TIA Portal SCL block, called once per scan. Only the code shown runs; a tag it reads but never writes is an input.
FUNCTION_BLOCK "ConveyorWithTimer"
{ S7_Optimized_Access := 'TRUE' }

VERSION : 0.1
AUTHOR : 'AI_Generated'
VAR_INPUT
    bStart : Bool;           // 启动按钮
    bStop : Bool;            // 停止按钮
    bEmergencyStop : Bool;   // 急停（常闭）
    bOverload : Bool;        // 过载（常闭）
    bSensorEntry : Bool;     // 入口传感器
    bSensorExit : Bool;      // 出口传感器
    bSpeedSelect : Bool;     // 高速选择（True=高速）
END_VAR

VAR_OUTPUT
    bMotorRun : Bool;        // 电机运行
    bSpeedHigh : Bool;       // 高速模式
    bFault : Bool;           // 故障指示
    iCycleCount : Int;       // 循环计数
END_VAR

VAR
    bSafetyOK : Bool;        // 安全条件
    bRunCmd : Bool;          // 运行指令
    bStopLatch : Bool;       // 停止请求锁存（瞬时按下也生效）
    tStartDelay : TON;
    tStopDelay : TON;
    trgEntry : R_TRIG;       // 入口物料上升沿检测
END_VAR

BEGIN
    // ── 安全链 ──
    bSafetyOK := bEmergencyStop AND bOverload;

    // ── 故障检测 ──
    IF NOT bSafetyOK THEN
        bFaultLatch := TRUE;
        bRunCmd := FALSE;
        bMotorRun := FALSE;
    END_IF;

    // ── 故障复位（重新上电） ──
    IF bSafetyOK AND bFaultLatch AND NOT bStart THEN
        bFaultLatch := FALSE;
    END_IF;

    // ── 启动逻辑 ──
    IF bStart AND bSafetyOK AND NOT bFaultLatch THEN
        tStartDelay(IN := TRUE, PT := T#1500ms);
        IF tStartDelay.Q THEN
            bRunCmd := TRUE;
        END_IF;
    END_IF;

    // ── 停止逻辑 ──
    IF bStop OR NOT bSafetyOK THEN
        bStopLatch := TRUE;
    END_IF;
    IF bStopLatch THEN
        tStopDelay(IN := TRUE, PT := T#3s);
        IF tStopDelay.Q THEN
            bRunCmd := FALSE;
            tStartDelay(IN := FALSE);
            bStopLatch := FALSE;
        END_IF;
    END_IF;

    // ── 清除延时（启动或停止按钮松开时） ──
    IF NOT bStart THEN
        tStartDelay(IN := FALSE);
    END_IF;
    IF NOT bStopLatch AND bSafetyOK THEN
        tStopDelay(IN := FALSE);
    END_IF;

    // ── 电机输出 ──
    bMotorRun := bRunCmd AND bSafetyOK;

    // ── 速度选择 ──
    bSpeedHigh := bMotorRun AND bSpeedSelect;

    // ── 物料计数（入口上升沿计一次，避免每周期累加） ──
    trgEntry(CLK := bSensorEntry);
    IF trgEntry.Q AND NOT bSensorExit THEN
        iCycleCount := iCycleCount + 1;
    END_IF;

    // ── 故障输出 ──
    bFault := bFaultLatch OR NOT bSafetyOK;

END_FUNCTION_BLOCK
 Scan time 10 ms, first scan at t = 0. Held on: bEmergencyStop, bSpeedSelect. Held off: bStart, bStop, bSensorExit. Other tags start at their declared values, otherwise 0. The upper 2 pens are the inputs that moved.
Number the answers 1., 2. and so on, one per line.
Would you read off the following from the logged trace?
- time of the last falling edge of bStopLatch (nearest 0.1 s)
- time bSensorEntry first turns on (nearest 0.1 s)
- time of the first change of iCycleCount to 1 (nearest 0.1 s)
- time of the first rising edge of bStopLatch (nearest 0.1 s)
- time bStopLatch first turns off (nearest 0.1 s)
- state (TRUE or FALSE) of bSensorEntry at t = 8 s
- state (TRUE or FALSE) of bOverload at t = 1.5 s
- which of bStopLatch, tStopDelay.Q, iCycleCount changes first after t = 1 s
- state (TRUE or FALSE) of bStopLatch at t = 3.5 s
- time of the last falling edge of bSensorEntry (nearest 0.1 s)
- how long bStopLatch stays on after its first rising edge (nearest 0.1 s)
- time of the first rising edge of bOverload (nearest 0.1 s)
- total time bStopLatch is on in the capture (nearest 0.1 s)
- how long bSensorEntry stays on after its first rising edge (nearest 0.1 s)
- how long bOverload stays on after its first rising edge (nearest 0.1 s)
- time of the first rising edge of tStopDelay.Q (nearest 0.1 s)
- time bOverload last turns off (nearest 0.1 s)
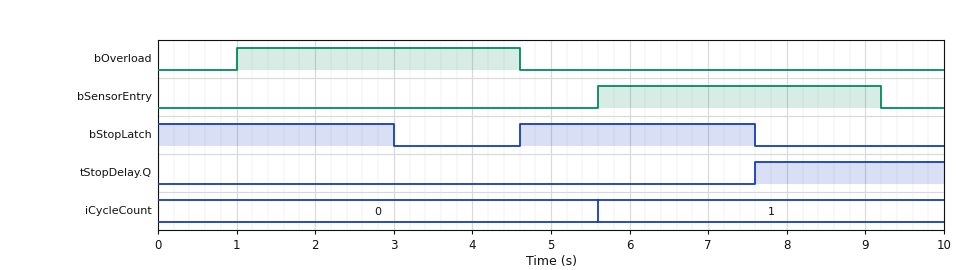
1. 7.6 s
2. 5.6 s
3. 5.6 s
4. 4.6 s
5. 3.0 s
6. TRUE
7. TRUE
8. bStopLatch
9. FALSE
10. 9.2 s
11. 3.0 s
12. 1.0 s
13. 6.0 s
14. 3.6 s
15. 3.6 s
16. 7.6 s
17. 4.6 s
